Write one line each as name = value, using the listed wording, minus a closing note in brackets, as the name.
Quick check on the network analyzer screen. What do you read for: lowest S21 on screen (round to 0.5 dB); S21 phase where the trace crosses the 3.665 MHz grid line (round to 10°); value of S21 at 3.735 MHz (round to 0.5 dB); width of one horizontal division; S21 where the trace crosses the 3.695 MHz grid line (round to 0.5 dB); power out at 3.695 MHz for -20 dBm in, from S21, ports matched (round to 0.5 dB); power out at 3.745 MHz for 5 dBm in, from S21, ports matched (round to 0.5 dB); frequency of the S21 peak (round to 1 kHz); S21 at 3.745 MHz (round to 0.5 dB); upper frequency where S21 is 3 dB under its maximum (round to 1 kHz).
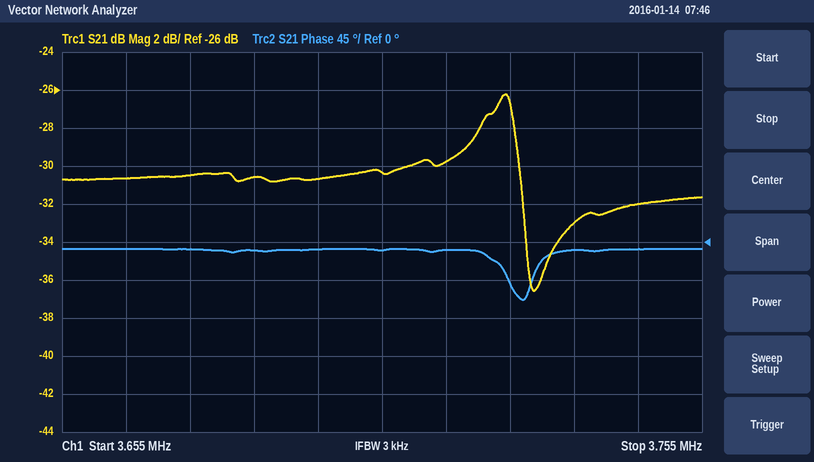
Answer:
lowest S21 on screen = -36.5 dB
S21 phase where the trace crosses the 3.665 MHz grid line = -10°
value of S21 at 3.735 MHz = -33.0 dB
width of one horizontal division = 10 kHz
S21 where the trace crosses the 3.695 MHz grid line = -30.5 dB
power out at 3.695 MHz for -20 dBm in, from S21, ports matched = -50.5 dBm
power out at 3.745 MHz for 5 dBm in, from S21, ports matched = -27.0 dBm
frequency of the S21 peak = 3.724 MHz
S21 at 3.745 MHz = -32.0 dB
upper frequency where S21 is 3 dB under its maximum = 3.726 MHz
